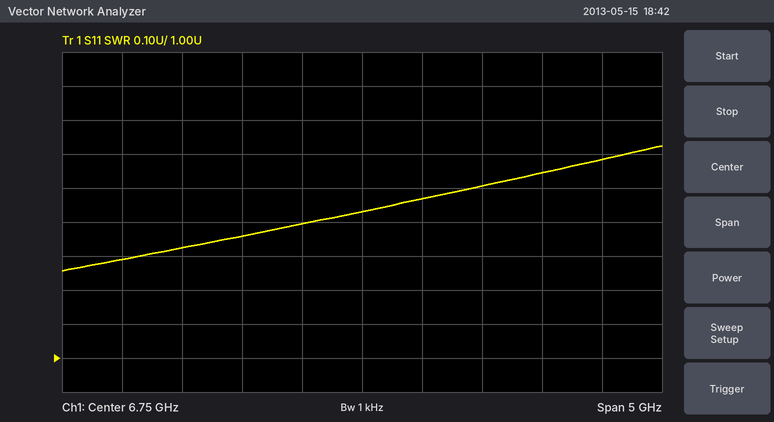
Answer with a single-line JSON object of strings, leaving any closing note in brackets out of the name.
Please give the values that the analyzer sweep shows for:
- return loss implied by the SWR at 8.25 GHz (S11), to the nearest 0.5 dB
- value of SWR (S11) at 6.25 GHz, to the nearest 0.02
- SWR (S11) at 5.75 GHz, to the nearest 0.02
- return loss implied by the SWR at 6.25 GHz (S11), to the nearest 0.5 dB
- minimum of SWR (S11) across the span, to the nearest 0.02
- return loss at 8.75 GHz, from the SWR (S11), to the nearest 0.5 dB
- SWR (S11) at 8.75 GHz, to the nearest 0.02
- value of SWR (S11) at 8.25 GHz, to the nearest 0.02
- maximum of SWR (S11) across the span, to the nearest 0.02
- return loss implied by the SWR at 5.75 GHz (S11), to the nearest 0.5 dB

{"return loss implied by the SWR at 8.25 GHz (S11), to the nearest 0.5 dB": "13.5 dB", "value of SWR (S11) at 6.25 GHz, to the nearest 0.02": "1.40", "SWR (S11) at 5.75 GHz, to the nearest 0.02": "1.36", "return loss implied by the SWR at 6.25 GHz (S11), to the nearest 0.5 dB": "15.5 dB", "minimum of SWR (S11) across the span, to the nearest 0.02": "1.26", "return loss at 8.75 GHz, from the SWR (S11), to the nearest 0.5 dB": "13.0 dB", "SWR (S11) at 8.75 GHz, to the nearest 0.02": "1.58", "value of SWR (S11) at 8.25 GHz, to the nearest 0.02": "1.54", "maximum of SWR (S11) across the span, to the nearest 0.02": "1.62", "return loss implied by the SWR at 5.75 GHz (S11), to the nearest 0.5 dB": "16.5 dB"}
